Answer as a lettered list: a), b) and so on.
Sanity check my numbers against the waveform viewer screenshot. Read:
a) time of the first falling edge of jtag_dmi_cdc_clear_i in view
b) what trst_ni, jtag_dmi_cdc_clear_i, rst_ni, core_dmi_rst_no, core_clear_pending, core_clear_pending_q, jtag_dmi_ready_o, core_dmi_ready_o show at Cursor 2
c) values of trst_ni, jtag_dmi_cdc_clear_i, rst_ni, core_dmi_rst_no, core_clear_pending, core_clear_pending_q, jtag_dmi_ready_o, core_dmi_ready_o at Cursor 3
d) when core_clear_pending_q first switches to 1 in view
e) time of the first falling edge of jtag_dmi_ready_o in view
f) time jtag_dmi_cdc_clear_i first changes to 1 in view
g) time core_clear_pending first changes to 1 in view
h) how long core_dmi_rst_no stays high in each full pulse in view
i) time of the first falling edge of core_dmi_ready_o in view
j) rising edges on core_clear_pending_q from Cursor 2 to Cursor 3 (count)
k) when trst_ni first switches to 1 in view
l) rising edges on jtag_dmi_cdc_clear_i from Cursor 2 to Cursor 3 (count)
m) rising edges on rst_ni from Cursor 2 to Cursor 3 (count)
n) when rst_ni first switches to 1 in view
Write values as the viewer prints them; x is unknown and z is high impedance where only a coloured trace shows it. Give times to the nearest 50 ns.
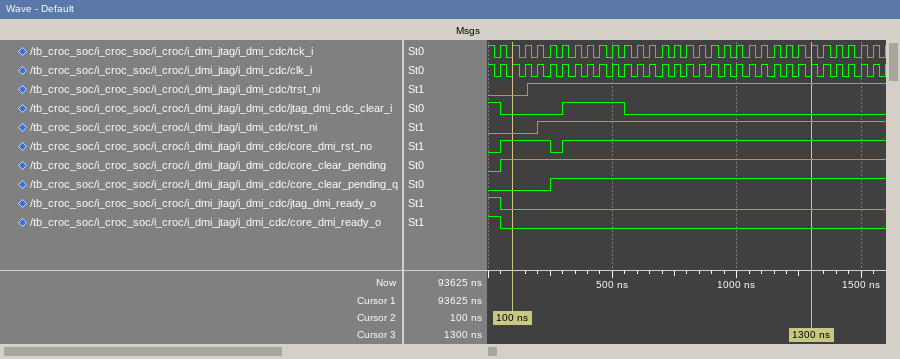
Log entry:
a) 50 ns
b) trst_ni=0, jtag_dmi_cdc_clear_i=0, rst_ni=0, core_dmi_rst_no=1, core_clear_pending=1, core_clear_pending_q=0, jtag_dmi_ready_o=0, core_dmi_ready_o=0
c) trst_ni=1, jtag_dmi_cdc_clear_i=0, rst_ni=1, core_dmi_rst_no=1, core_clear_pending=1, core_clear_pending_q=1, jtag_dmi_ready_o=0, core_dmi_ready_o=0
d) 250 ns
e) 50 ns
f) 300 ns
g) 50 ns
h) 200 ns
i) 50 ns
j) 1
k) 150 ns
l) 1
m) 1
n) 200 ns
